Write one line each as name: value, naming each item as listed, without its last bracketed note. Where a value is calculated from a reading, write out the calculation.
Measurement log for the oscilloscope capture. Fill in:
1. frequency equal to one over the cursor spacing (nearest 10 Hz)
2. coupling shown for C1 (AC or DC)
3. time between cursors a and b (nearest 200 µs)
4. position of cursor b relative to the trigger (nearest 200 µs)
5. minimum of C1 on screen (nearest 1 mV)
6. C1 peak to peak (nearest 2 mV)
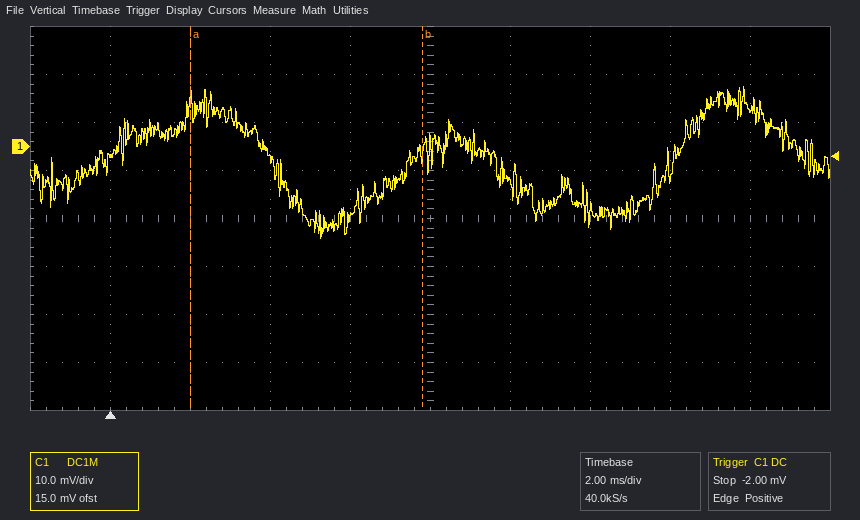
frequency equal to one over the cursor spacing: 1 / 5.8 ms ≈ 170 Hz
coupling shown for C1: DC
time between cursors a and b: 5.8 ms
position of cursor b relative to the trigger: +7.8 ms
minimum of C1 on screen: -19 mV
C1 peak to peak: 32 mV
